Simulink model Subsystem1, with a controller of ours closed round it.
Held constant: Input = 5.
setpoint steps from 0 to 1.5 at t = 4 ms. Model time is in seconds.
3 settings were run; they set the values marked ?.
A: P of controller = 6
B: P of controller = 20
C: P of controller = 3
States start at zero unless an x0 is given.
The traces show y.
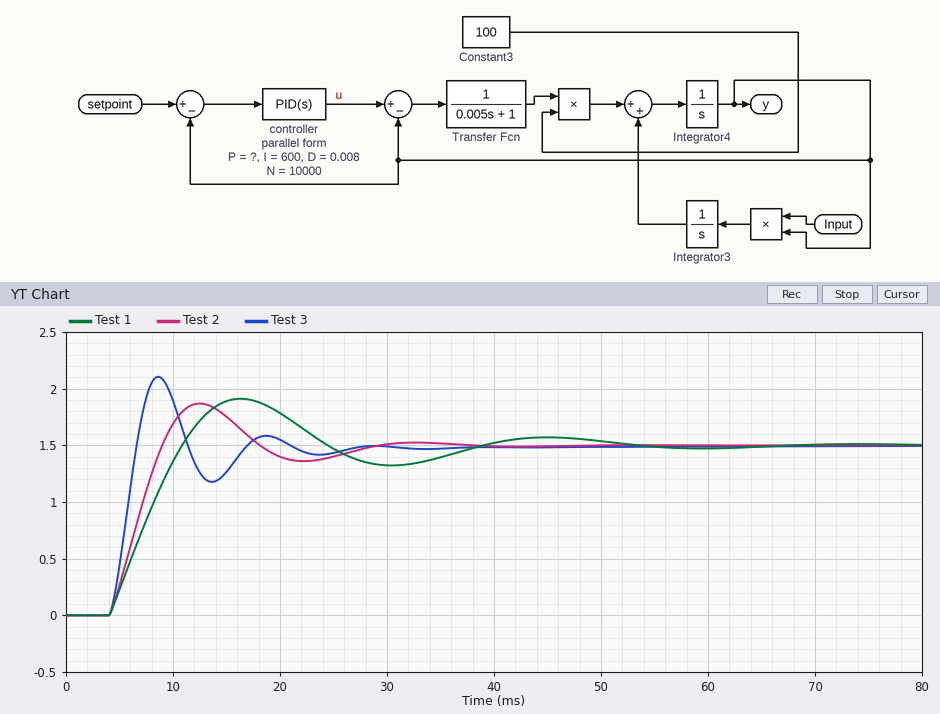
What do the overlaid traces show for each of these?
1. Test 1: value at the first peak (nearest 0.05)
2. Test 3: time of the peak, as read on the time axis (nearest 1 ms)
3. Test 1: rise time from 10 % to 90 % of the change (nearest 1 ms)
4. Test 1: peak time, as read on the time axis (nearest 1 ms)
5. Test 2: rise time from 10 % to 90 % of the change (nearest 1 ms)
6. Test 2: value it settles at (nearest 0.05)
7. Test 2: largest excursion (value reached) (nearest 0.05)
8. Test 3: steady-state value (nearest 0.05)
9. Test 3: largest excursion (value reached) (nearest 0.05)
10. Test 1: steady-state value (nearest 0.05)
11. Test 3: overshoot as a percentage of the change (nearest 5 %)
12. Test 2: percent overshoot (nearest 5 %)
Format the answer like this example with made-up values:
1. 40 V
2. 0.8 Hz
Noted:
1. 1.90
2. 9 ms
3. 5 ms
4. 16 ms
5. 4 ms
6. 1.50
7. 1.85
8. 1.50
9. 2.10
10. 1.50
11. 40 %
12. 25 %
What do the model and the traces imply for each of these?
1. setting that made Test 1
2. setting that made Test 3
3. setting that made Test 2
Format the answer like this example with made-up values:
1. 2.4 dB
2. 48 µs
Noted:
1. C
2. B
3. A
